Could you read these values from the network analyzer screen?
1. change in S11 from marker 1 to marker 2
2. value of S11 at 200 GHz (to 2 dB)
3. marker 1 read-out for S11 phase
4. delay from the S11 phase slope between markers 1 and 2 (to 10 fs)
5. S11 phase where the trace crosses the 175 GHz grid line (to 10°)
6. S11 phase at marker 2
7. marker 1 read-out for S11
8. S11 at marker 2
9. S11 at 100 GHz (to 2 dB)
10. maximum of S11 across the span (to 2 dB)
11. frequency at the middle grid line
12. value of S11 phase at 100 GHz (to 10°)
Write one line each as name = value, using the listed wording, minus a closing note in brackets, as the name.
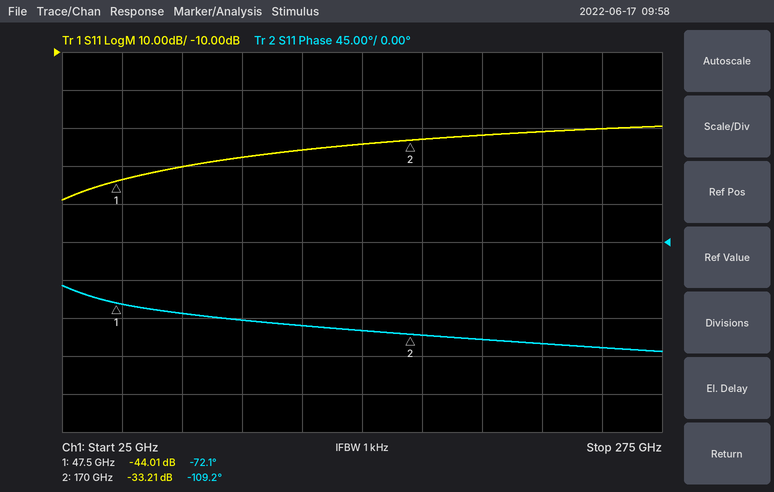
change in S11 from marker 1 to marker 2 = 10.80 dB
value of S11 at 200 GHz = -32 dB
marker 1 read-out for S11 phase = -72.1°
delay from the S11 phase slope between markers 1 and 2 = 840 fs
S11 phase where the trace crosses the 175 GHz grid line = -110°
S11 phase at marker 2 = -109.2°
marker 1 read-out for S11 = -44.01 dB
S11 at marker 2 = -33.21 dB
S11 at 100 GHz = -38 dB
maximum of S11 across the span = -30 dB
frequency at the middle grid line = 150 GHz
value of S11 phase at 100 GHz = -90°
